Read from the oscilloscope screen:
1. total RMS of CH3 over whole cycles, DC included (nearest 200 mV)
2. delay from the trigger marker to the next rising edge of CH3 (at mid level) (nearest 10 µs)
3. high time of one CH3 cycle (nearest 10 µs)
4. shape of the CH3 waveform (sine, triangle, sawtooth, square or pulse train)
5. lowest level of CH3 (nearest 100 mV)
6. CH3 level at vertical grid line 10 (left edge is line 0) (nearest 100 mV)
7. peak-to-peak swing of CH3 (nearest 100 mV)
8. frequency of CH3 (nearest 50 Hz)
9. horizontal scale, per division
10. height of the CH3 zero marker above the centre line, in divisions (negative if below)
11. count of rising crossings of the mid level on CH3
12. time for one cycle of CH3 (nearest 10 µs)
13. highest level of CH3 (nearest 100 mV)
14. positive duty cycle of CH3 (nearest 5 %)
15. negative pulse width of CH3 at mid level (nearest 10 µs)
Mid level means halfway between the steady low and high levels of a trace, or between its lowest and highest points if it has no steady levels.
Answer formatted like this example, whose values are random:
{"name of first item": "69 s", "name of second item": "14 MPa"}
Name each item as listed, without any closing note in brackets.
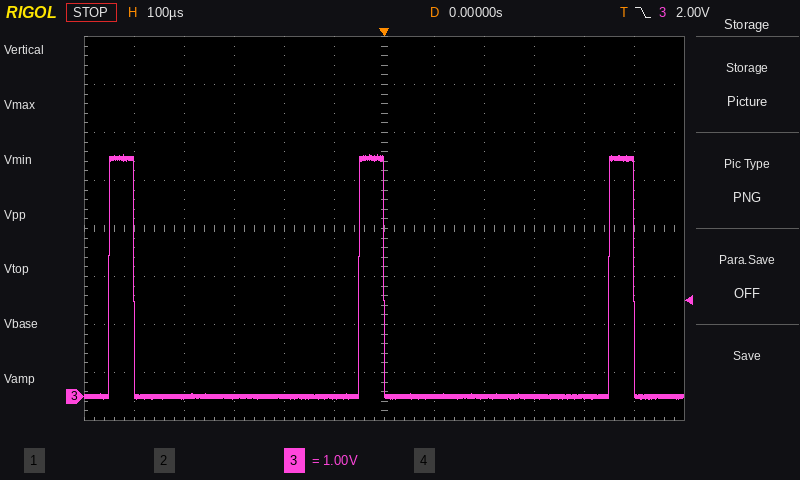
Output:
{"total RMS of CH3 over whole cycles, DC included": "1.6 V", "delay from the trigger marker to the next rising edge of CH3 (at mid level)": "450 µs", "high time of one CH3 cycle": "50 µs", "shape of the CH3 waveform": "pulse train", "lowest level of CH3": "-100 mV", "CH3 level at vertical grid line 10 (left edge is line 0)": "0.0 V", "peak-to-peak swing of CH3": "5.1 V", "frequency of CH3": "2.00 kHz", "horizontal scale, per division": "100 µs", "height of the CH3 zero marker above the centre line, in divisions": "-3.5 div", "count of rising crossings of the mid level on CH3": "3", "time for one cycle of CH3": "500 µs", "highest level of CH3": "5.0 V", "positive duty cycle of CH3": "10 %", "negative pulse width of CH3 at mid level": "450 µs"}
